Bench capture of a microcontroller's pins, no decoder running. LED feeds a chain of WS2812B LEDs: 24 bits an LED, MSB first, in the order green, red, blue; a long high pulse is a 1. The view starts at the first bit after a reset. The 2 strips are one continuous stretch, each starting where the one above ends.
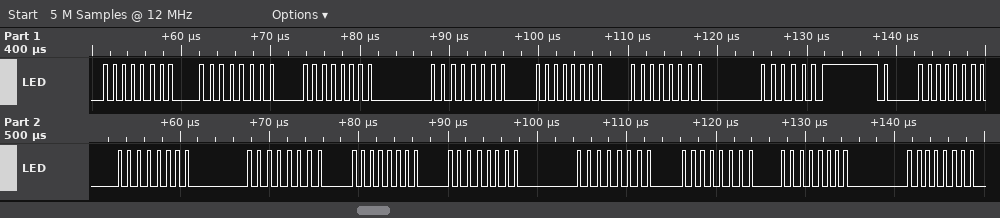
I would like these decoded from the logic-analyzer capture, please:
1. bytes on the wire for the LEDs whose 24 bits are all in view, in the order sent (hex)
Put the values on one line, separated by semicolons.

00 00 00 00 00 00 02 00 00 00 00 00 00 00 00
